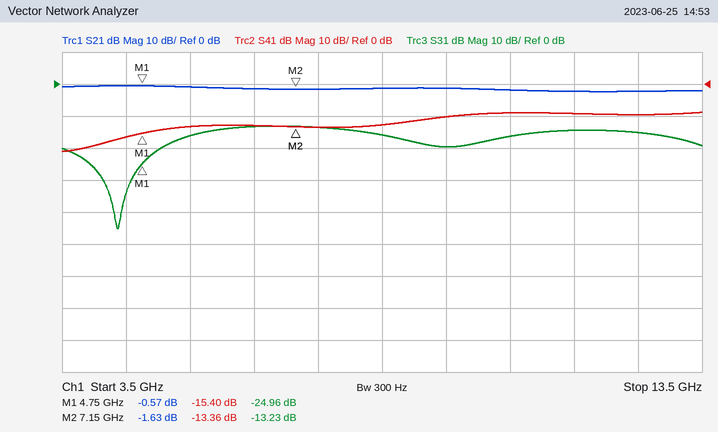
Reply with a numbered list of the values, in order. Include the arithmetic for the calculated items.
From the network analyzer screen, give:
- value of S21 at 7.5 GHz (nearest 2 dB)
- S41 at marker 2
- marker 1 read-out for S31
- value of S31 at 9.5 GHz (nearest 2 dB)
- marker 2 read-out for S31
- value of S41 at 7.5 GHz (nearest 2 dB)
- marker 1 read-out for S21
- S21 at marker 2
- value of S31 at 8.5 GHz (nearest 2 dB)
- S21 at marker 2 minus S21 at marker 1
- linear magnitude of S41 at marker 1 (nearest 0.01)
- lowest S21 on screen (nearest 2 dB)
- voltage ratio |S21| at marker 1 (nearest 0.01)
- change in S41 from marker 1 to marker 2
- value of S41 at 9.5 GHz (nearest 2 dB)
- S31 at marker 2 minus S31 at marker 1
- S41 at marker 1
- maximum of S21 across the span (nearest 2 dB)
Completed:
1. -2 dB
2. -13.36 dB
3. -24.96 dB
4. -20 dB
5. -13.23 dB
6. -14 dB
7. -0.57 dB
8. -1.63 dB
9. -16 dB
10. -1.63 − (-0.57) = -1.06 dB
11. 10^(-15.4/20) ≈ 0.17
12. -2 dB
13. 10^(-0.57/20) ≈ 0.94
14. -13.36 − (-15.4) = 2.04 dB
15. -10 dB
16. -13.23 − (-24.96) = 11.73 dB
17. -15.40 dB
18. 0 dB
